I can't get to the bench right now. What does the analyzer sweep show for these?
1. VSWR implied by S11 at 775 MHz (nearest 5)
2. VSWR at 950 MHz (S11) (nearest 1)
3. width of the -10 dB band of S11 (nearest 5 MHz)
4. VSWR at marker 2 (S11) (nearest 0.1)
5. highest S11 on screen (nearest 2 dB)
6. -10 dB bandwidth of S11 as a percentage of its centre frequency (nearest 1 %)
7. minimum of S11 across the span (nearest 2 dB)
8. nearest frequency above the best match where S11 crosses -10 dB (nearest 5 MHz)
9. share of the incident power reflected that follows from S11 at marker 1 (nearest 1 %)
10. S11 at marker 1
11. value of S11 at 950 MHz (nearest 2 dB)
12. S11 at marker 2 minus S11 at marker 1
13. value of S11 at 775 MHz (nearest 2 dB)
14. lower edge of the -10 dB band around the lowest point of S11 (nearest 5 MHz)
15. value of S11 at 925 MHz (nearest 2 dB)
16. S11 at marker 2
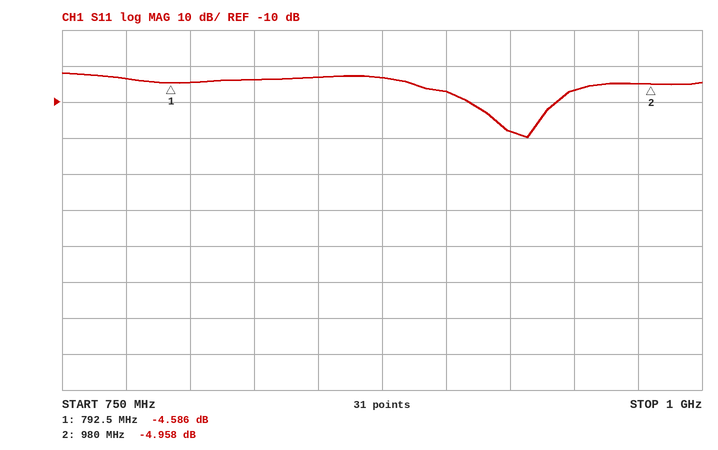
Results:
5
3
35 MHz
3.6
-2 dB
4 %
-20 dB
945 MHz
35 %
-4.586 dB
-6 dB
-0.372 dB
-4 dB
910 MHz
-18 dB
-4.958 dB
